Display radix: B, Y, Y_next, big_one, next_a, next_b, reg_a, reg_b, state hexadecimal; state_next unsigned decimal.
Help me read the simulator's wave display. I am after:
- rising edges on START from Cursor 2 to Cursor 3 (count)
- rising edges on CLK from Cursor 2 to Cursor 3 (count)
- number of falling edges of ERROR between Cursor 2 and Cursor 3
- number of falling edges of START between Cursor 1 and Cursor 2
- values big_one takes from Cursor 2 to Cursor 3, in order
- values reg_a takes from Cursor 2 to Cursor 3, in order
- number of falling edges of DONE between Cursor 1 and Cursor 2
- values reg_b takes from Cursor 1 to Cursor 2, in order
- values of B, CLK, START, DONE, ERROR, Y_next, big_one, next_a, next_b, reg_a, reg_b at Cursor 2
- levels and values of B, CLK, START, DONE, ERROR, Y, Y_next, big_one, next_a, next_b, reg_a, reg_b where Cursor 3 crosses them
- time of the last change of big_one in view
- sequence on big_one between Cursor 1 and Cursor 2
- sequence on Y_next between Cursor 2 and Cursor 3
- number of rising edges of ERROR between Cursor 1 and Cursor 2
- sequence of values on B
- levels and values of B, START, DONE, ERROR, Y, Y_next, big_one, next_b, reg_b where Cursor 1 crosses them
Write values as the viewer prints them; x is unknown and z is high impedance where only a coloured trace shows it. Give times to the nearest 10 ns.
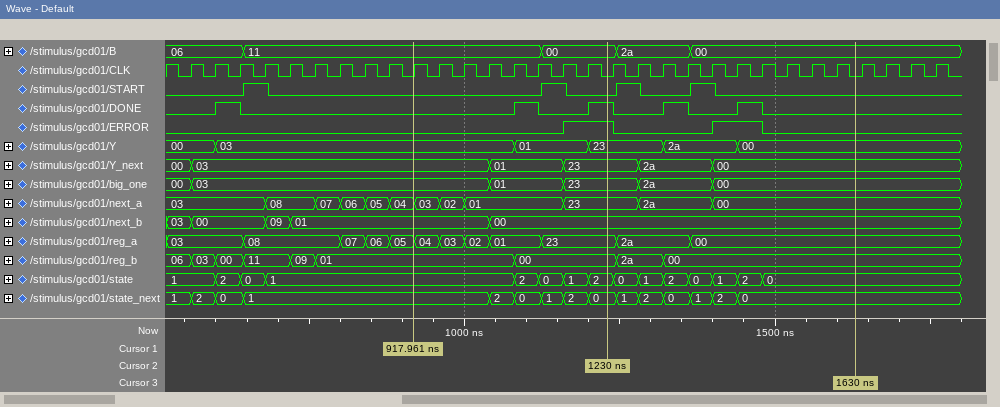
2
10
2
1
23, 2a, 00
23, 2a, 00
1
01, 00
B=00, CLK=0, START=0, DONE=1, ERROR=1, Y_next=23, big_one=23, next_a=23, next_b=00, reg_a=23, reg_b=00
B=00, CLK=0, START=0, DONE=0, ERROR=0, Y=00, Y_next=00, big_one=00, next_a=00, next_b=00, reg_a=00, reg_b=00
1400 ns
03, 01, 23
23, 2a, 00
1
06, 11, 00, 2a, 00
B=11, START=0, DONE=0, ERROR=0, Y=03, Y_next=03, big_one=03, next_b=01, reg_b=01
